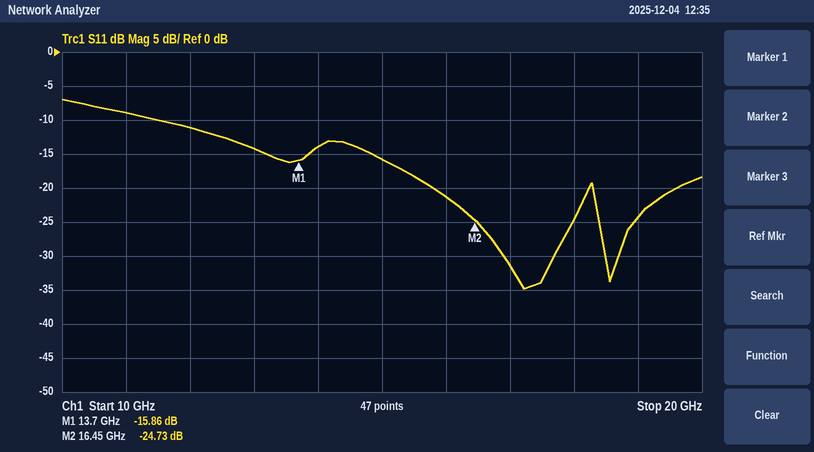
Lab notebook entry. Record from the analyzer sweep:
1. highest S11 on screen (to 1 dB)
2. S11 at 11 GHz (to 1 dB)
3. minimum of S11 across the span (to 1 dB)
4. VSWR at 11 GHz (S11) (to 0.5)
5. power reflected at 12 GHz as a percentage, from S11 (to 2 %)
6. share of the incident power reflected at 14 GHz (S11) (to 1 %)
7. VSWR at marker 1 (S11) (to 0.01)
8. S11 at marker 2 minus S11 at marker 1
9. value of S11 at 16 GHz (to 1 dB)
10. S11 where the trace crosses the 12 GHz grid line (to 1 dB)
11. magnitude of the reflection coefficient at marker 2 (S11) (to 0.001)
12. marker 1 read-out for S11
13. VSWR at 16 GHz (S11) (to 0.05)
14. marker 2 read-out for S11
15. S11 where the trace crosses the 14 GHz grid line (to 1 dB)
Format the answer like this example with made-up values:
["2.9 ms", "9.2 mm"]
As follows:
["-7 dB", "-9 dB", "-35 dB", "2.0", "8 %", "4 %", "1.38", "-8.87 dB", "-21 dB", "-11 dB", "0.058", "-15.86 dB", "1.20", "-24.73 dB", "-14 dB"]
